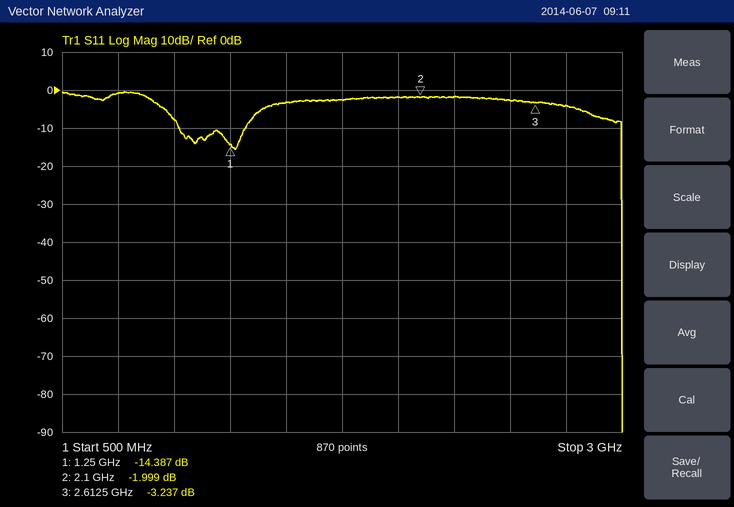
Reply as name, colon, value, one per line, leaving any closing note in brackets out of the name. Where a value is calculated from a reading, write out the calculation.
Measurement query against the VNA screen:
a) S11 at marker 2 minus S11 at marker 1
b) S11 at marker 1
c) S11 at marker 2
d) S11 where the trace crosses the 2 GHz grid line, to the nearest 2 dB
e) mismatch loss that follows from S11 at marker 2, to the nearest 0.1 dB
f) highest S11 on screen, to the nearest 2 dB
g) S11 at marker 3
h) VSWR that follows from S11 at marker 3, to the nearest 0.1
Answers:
S11 at marker 2 minus S11 at marker 1: -1.999 − (-14.387) = 12.388 dB
S11 at marker 1: -14.387 dB
S11 at marker 2: -1.999 dB
S11 where the trace crosses the 2 GHz grid line, to the nearest 2 dB: -2 dB
mismatch loss that follows from S11 at marker 2, to the nearest 0.1 dB: −10 log10(1 − 10^(-1.999/10)) ≈ 4.3 dB
highest S11 on screen, to the nearest 2 dB: 0 dB
S11 at marker 3: -3.237 dB
VSWR that follows from S11 at marker 3, to the nearest 0.1: (1 + 0.6889)/(1 − 0.6889) ≈ 5.4
